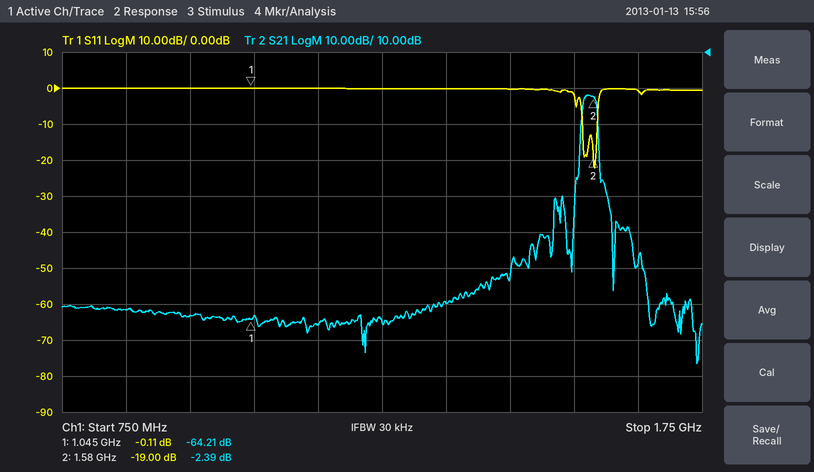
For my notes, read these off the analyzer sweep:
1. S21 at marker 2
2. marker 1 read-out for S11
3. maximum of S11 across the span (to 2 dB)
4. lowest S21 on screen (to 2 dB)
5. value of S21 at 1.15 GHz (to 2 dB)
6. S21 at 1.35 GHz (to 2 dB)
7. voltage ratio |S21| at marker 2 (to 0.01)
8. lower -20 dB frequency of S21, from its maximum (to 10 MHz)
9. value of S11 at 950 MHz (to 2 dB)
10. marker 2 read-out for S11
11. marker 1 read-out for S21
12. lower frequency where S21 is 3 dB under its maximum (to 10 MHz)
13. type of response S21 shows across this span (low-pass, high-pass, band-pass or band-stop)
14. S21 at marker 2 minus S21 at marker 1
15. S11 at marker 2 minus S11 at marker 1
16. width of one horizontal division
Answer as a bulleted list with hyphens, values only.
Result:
- -2.39 dB
- -0.11 dB
- 0 dB
- -76 dB
- -66 dB
- -60 dB
- 0.76
- 1.56 GHz
- 0 dB
- -19.00 dB
- -64.21 dB
- 1.56 GHz
- band-pass
- 61.82 dB
- -18.89 dB
- 100 MHz
